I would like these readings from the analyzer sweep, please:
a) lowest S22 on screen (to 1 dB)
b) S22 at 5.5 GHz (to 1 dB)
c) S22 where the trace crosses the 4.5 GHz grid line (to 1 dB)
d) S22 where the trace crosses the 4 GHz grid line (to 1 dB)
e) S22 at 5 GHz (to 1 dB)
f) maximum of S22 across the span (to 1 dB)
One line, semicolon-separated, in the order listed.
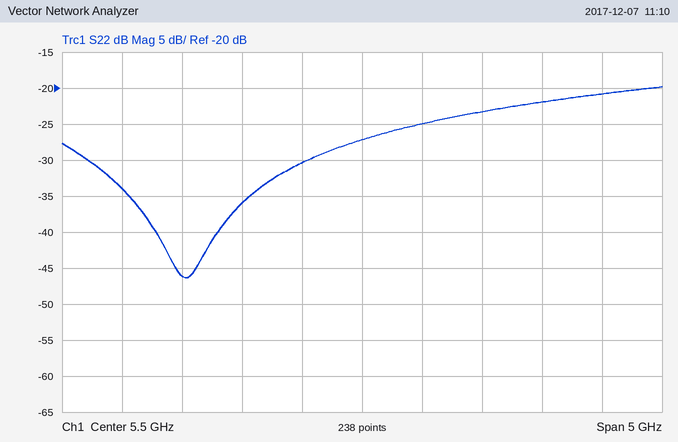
-46 dB; -27 dB; -36 dB; -46 dB; -30 dB; -20 dB
